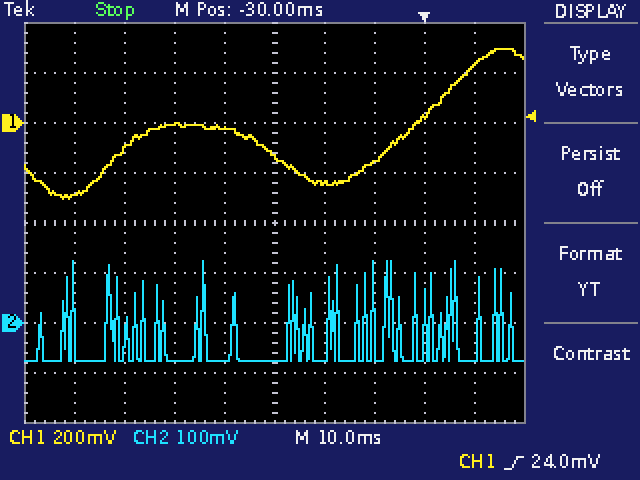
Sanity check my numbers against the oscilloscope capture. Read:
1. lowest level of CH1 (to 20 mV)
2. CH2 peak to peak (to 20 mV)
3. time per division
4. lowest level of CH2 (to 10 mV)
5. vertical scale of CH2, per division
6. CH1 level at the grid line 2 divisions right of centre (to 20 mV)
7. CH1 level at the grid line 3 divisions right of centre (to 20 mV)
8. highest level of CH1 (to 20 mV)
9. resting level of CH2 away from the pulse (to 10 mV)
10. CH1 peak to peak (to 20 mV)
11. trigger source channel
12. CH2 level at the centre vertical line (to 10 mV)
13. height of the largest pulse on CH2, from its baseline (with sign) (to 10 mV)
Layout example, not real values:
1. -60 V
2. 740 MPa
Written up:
1. -300 mV
2. 200 mV
3. 10 ms
4. -80 mV
5. 100 mV
6. -160 mV
7. 20 mV
8. 300 mV
9. -80 mV
10. 600 mV
11. CH1
12. -80 mV
13. +200 mV
